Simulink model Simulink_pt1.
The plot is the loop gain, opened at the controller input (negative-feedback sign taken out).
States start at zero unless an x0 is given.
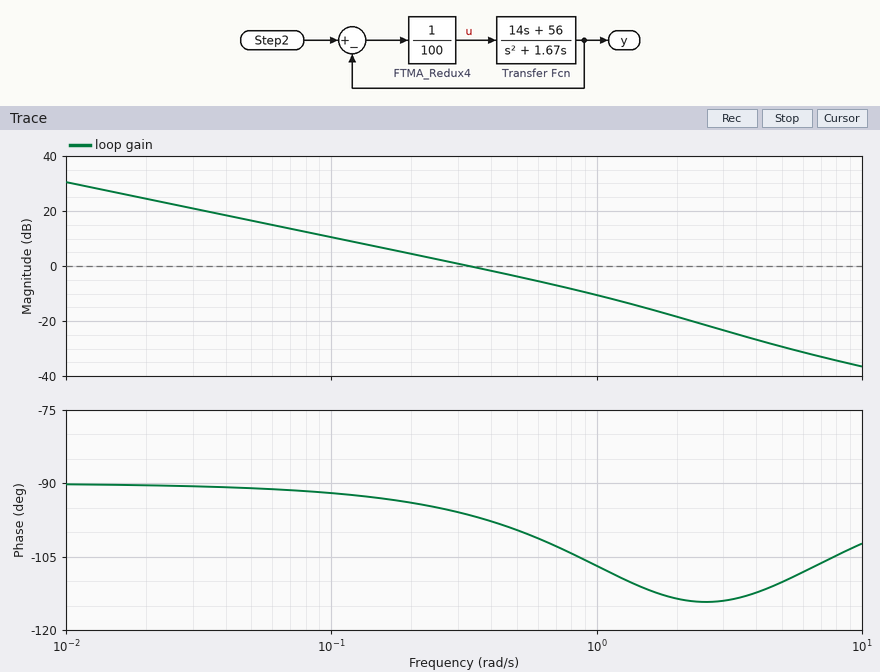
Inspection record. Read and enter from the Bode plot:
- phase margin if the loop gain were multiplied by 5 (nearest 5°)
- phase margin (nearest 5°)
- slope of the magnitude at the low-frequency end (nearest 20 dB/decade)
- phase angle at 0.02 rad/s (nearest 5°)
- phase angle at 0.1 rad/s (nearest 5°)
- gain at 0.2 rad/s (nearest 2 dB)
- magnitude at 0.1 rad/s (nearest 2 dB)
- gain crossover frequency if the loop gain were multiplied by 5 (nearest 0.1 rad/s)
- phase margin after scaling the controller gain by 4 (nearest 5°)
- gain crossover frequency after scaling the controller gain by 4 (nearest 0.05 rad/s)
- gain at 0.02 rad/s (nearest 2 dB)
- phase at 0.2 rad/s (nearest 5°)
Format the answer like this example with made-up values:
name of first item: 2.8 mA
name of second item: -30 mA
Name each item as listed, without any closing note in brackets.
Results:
phase margin if the loop gain were multiplied by 5: 70°
phase margin: 85°
slope of the magnitude at the low-frequency end: -20 dB/decade
phase angle at 0.02 rad/s: -90°
phase angle at 0.1 rad/s: -90°
gain at 0.2 rad/s: 4 dB
magnitude at 0.1 rad/s: 10 dB
gain crossover frequency if the loop gain were multiplied by 5: 1.4 rad/s
phase margin after scaling the controller gain by 4: 70°
gain crossover frequency after scaling the controller gain by 4: 1.15 rad/s
gain at 0.02 rad/s: 24 dB
phase at 0.2 rad/s: -95°
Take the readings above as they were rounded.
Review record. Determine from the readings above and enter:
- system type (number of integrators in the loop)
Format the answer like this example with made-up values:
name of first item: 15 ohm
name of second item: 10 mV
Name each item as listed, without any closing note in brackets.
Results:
system type: 1
